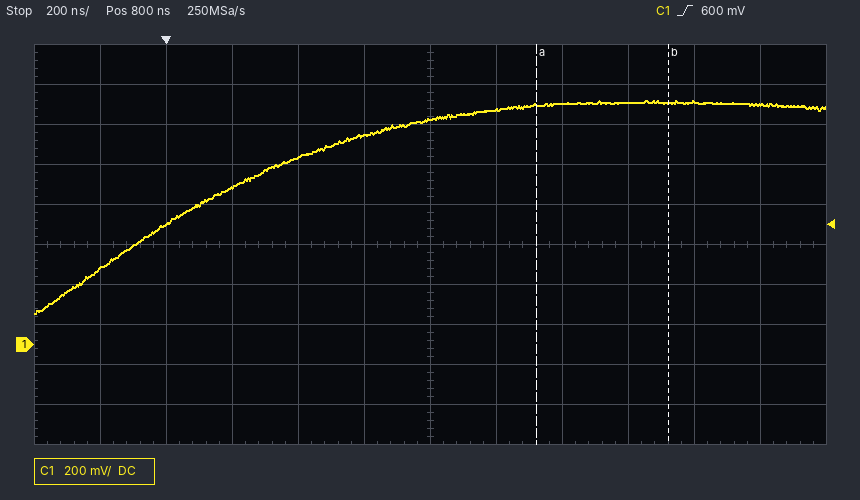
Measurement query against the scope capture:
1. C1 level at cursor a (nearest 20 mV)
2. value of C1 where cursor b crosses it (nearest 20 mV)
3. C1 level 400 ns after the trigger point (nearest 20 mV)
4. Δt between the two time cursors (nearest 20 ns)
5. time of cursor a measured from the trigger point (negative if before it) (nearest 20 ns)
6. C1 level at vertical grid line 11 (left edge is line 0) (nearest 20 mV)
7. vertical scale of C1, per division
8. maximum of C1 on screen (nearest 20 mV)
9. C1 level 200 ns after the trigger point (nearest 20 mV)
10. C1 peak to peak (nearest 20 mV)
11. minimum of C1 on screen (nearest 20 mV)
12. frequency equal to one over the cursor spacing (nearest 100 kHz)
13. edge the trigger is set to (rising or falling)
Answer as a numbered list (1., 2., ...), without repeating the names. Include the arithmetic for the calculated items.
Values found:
1. 1.20 V
2. 1.20 V
3. 940 mV
4. 400 ns
5. +1.12 µs
6. 1.20 V
7. 200 mV
8. 1.22 V
9. 780 mV
10. 1.22 V − (160 mV) = 1.06 V
11. 160 mV
12. 1 / 400 ns ≈ 2.5 MHz
13. rising
